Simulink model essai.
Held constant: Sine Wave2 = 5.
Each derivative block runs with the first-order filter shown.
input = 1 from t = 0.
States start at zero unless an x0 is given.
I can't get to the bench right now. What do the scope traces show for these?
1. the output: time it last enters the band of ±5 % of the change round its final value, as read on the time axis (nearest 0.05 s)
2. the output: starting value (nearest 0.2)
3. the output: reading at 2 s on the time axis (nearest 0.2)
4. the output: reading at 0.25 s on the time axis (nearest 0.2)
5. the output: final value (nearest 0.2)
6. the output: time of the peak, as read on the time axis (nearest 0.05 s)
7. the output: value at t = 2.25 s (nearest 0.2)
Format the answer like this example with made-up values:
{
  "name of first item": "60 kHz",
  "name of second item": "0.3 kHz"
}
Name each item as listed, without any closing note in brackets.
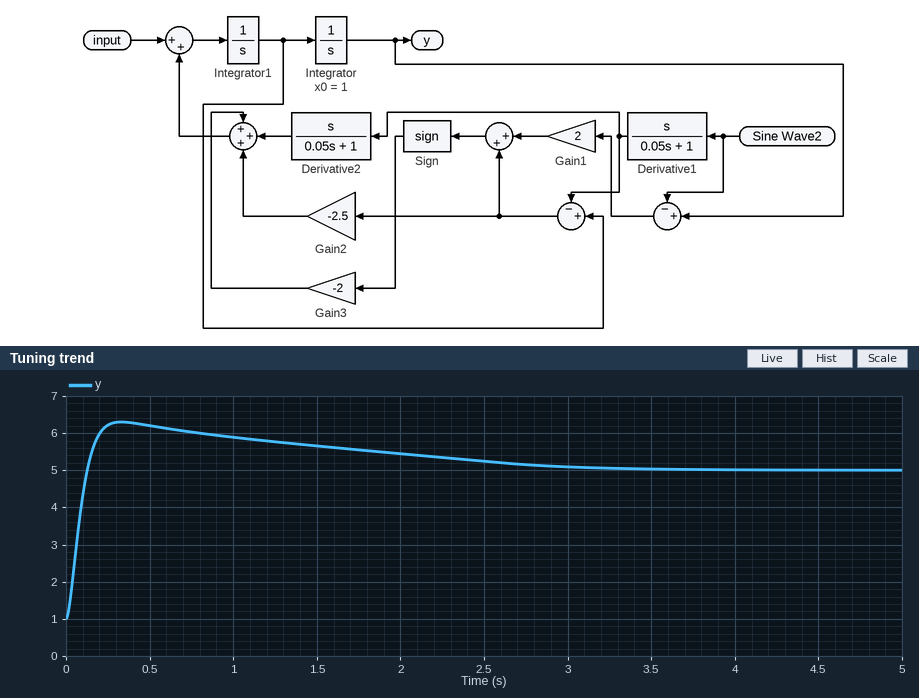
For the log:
{
  "the output: time it last enters the band of ±5 % of the change round its final value, as read on the time axis": "2.60 s",
  "the output: starting value": "1.0",
  "the output: reading at 2 s on the time axis": "5.4",
  "the output: reading at 0.25 s on the time axis": "6.2",
  "the output: final value": "5.0",
  "the output: time of the peak, as read on the time axis": "0.35 s",
  "the output: value at t = 2.25 s": "5.4"
}
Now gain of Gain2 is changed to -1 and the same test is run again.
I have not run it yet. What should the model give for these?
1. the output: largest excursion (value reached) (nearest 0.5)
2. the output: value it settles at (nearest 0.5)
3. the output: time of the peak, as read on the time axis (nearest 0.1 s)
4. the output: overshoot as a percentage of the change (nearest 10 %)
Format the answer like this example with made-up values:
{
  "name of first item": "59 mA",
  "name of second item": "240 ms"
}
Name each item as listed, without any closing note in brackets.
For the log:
{
  "the output: largest excursion (value reached)": "6.0",
  "the output: value it settles at": "5.0",
  "the output: time of the peak, as read on the time axis": "0.4 s",
  "the output: overshoot as a percentage of the change": "30 %"
}
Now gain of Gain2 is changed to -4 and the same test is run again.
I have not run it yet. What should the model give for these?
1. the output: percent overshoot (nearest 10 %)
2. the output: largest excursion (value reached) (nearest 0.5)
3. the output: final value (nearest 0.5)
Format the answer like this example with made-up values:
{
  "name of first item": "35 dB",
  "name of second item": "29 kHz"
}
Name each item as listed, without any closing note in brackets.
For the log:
{
  "the output: percent overshoot": "30 %",
  "the output: largest excursion (value reached)": "6.5",
  "the output: final value": "5.0"
}
